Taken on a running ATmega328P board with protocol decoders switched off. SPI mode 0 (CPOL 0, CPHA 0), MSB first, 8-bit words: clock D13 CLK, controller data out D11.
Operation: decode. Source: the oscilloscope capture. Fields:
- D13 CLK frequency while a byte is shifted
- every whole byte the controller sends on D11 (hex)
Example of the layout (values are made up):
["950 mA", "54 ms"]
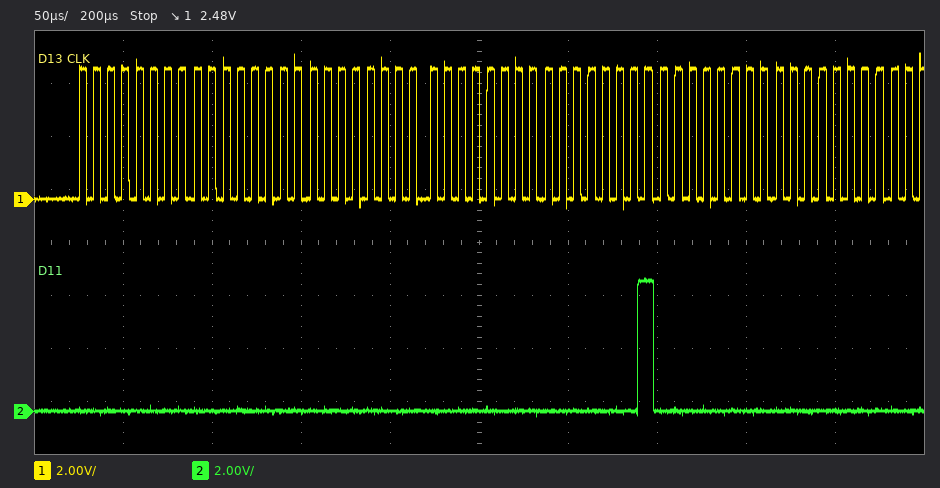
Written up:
["125 kHz", "00 00 00 00 01 00 00"]
